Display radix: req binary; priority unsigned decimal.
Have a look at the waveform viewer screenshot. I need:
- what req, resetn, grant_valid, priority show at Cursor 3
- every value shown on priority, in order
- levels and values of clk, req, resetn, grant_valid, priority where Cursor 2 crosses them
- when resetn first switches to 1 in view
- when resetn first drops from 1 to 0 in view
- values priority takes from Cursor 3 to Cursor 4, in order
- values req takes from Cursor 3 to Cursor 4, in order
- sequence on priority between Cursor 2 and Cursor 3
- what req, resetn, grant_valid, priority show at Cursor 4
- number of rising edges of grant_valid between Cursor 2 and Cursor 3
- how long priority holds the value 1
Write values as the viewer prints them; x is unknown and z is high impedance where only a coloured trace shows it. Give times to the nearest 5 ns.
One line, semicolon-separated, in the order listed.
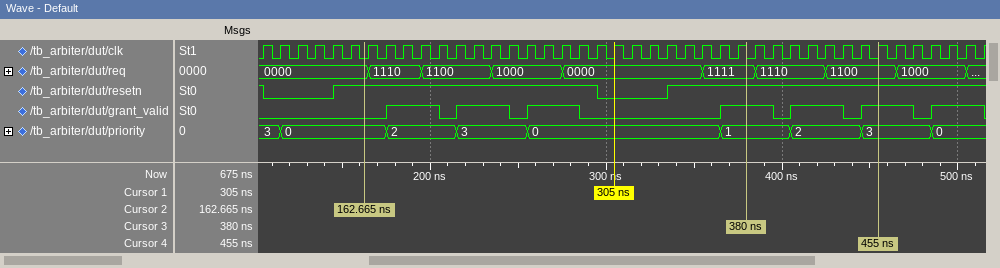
req=1111, resetn=1, grant_valid=1, priority=1; 3, 0, 2, 3, 0, 1, 2, 3, 0; clk=0, req=0000, resetn=1, grant_valid=0, priority=0; 145 ns; 105 ns; 1, 2, 3; 1111, 1110, 1100; 0, 2, 3, 0, 1; req=1100, resetn=1, grant_valid=1, priority=3; 4; 40 ns
